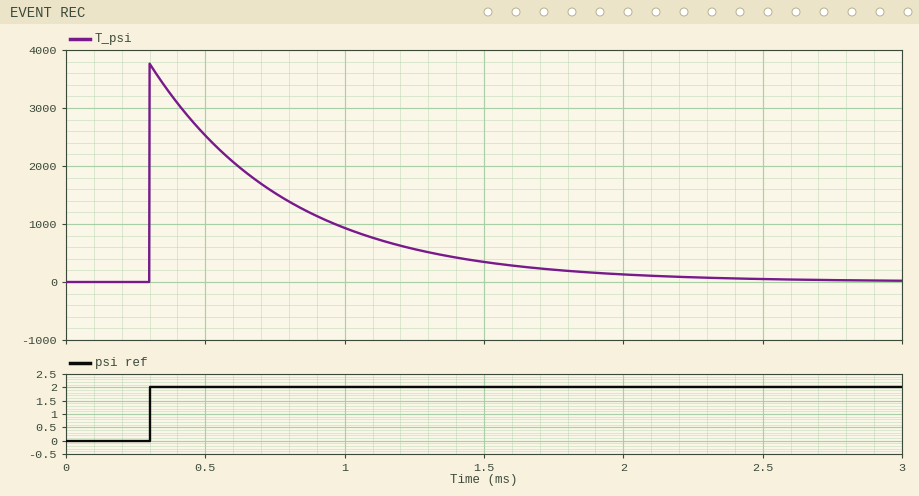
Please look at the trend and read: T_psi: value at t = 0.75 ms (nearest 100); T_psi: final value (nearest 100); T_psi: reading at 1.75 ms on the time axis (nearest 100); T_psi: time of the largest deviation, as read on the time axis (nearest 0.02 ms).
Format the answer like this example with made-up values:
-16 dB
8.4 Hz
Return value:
1500
0
200
0.30 ms
